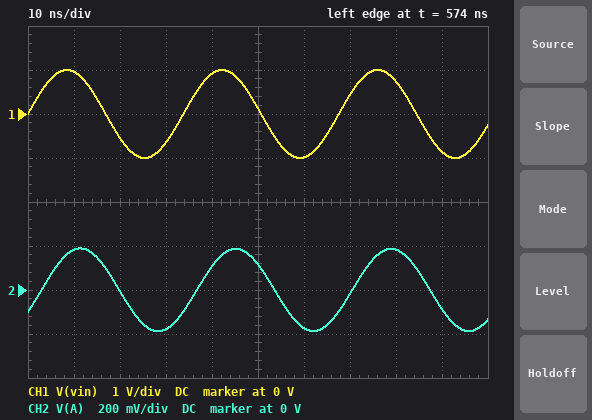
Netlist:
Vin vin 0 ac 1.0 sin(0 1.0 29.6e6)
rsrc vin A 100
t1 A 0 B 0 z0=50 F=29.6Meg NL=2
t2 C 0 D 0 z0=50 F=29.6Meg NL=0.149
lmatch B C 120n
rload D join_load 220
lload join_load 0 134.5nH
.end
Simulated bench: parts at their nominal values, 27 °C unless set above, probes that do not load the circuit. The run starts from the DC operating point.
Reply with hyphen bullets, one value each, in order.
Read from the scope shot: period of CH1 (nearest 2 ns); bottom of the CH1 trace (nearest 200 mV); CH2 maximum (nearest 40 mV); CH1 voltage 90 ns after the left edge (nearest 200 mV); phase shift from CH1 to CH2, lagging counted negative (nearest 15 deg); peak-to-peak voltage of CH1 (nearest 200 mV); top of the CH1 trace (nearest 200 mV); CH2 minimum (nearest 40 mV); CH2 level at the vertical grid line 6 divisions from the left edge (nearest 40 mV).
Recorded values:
- 34 ns
- -1.0 V
- 200 mV
- -800 mV
- -30 deg
- 2.0 V
- 1.0 V
- -200 mV
- -160 mV
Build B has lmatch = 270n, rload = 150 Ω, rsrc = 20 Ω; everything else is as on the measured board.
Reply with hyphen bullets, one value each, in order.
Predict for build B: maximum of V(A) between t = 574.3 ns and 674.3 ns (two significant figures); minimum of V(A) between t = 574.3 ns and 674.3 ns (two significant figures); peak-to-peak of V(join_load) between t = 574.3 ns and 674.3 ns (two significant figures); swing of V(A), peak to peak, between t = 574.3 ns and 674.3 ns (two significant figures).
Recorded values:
- 620 mV
- -620 mV
- 430 mV
- 1.2 V
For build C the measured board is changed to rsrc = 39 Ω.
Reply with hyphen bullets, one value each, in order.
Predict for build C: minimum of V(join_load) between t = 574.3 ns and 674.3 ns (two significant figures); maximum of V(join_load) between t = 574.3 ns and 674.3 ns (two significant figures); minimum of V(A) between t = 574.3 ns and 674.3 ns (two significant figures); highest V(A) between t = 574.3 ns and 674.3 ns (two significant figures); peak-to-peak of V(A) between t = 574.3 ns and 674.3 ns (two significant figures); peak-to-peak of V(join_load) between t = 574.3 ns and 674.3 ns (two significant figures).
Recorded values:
- -120 mV
- 120 mV
- -380 mV
- 380 mV
- 760 mV
- 240 mV
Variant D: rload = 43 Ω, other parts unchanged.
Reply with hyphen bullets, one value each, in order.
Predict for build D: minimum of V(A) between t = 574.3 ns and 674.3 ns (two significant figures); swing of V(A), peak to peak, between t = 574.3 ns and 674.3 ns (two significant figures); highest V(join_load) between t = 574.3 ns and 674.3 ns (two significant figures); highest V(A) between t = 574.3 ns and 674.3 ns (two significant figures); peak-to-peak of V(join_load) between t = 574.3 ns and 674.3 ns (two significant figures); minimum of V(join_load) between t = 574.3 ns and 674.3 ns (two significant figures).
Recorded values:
- -460 mV
- 910 mV
- 190 mV
- 460 mV
- 380 mV
- -190 mV
